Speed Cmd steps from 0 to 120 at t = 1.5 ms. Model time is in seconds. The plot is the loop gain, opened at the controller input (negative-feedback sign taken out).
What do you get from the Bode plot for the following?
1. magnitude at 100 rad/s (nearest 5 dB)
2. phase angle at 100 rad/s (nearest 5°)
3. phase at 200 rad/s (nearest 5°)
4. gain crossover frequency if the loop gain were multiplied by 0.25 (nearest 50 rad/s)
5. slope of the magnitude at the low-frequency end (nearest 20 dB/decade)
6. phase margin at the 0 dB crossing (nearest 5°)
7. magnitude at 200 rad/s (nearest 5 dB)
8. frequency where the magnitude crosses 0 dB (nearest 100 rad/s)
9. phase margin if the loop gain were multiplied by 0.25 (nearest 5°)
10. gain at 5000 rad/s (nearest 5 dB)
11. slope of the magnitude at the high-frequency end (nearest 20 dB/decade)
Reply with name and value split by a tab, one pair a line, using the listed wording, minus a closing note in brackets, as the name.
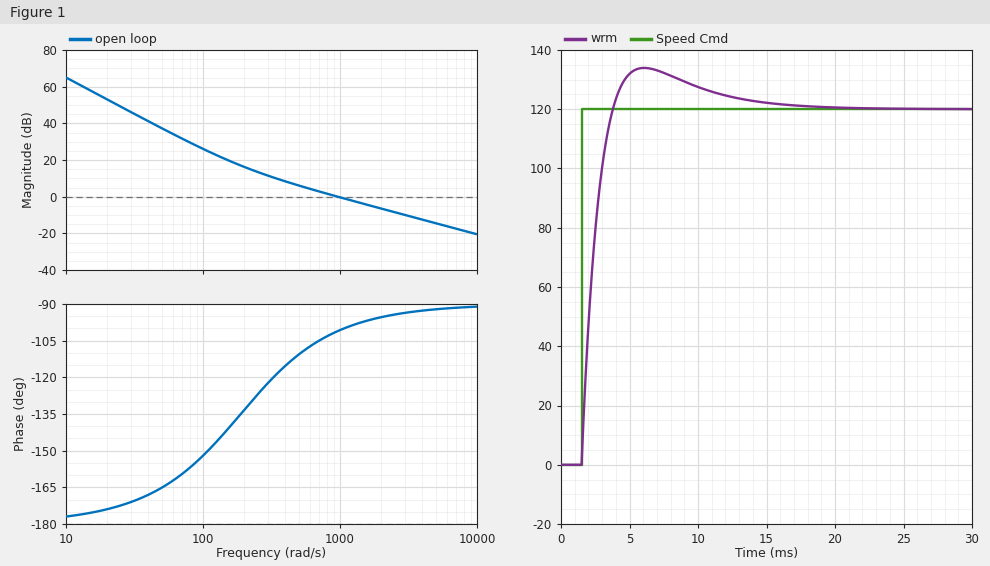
magnitude at 100 rad/s	25 dB
phase angle at 100 rad/s	-150°
phase at 200 rad/s	-135°
gain crossover frequency if the loop gain were multiplied by 0.25	300 rad/s
slope of the magnitude at the low-frequency end	-40 dB/decade
phase margin at the 0 dB crossing	80°
magnitude at 200 rad/s	15 dB
frequency where the magnitude crosses 0 dB	1000 rad/s
phase margin if the loop gain were multiplied by 0.25	55°
gain at 5000 rad/s	-15 dB
slope of the magnitude at the high-frequency end	-20 dB/decade
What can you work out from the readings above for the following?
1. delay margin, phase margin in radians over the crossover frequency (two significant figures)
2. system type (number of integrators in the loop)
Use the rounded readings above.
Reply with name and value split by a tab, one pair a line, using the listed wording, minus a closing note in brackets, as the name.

delay margin, phase margin in radians over the crossover frequency	0.0014 s
system type	2
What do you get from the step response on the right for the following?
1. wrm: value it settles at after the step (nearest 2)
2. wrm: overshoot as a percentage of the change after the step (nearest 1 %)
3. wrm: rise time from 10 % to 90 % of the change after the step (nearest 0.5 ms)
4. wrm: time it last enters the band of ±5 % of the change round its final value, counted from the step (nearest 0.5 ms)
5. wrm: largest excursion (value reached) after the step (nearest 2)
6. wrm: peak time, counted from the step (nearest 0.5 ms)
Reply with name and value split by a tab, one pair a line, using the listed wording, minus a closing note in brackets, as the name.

wrm: value it settles at after the step	120
wrm: overshoot as a percentage of the change after the step	12 %
wrm: rise time from 10 % to 90 % of the change after the step	1.5 ms
wrm: time it last enters the band of ±5 % of the change round its final value, counted from the step	9.5 ms
wrm: largest excursion (value reached) after the step	134
wrm: peak time, counted from the step	4.5 ms
